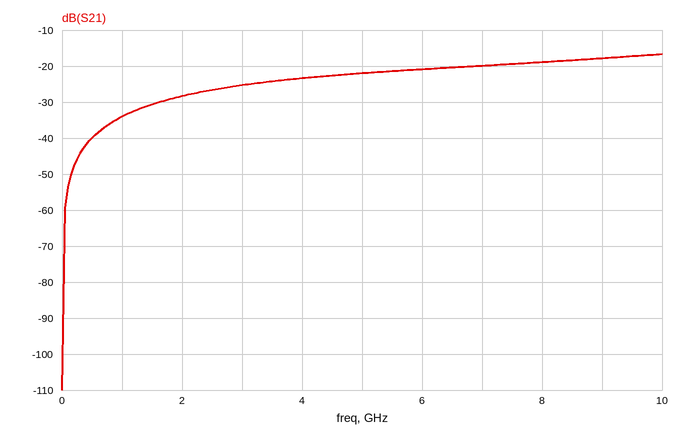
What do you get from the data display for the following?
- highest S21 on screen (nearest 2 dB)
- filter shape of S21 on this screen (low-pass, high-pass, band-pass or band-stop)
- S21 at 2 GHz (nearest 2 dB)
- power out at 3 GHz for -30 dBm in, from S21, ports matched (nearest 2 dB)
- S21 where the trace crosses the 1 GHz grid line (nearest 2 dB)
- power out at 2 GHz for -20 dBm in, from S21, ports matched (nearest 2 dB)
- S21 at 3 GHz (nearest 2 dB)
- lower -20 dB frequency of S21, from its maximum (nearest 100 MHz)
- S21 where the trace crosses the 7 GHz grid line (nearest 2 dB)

-16 dB
high-pass
-28 dB
-56 dBm
-34 dB
-48 dBm
-26 dB
700 MHz
-20 dB
